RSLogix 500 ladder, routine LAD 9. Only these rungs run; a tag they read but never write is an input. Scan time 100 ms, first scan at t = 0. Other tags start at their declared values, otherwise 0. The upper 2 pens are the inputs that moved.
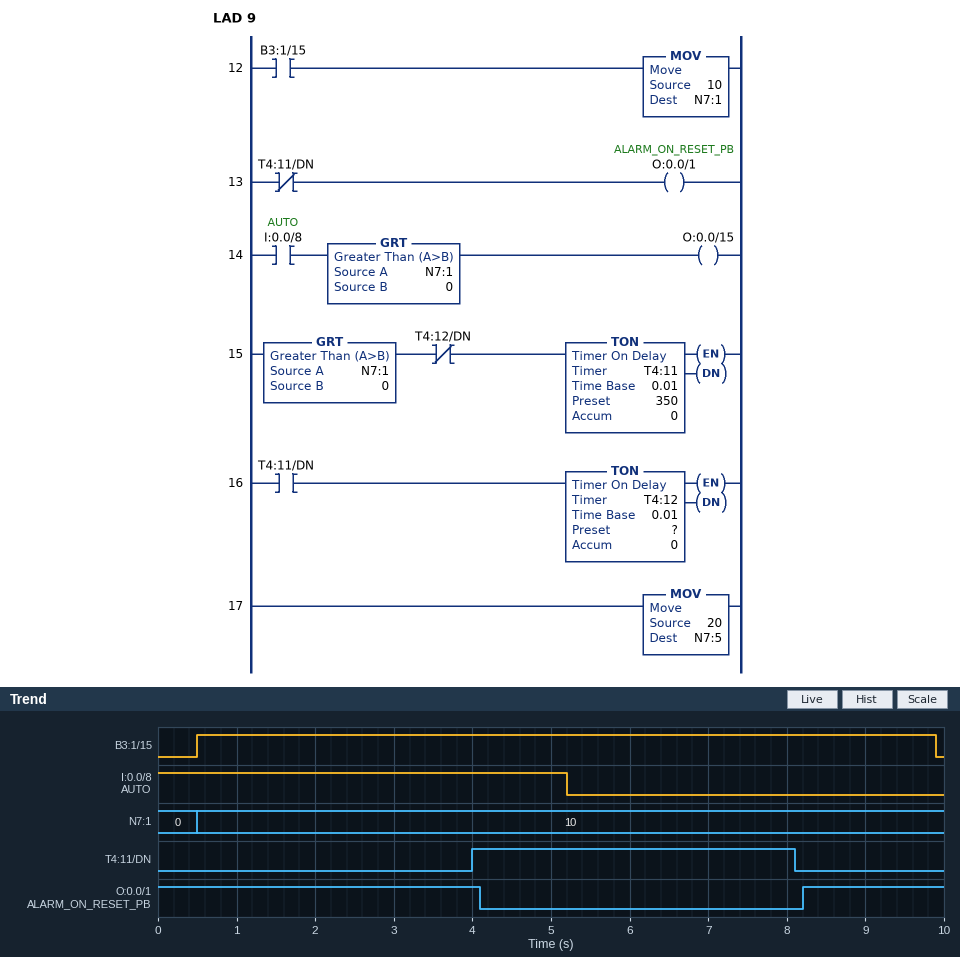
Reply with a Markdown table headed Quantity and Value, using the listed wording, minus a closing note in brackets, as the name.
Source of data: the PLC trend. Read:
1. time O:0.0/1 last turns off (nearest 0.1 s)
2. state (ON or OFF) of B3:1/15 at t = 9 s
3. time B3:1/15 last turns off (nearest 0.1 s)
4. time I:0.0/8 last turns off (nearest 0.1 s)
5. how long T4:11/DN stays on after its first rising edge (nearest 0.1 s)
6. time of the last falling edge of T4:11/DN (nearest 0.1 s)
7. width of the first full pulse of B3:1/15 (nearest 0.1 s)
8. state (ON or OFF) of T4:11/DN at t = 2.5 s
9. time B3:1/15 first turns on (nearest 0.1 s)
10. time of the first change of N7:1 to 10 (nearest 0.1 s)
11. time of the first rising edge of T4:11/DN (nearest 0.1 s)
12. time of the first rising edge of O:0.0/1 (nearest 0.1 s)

| Quantity | Value |
|---|---|
| time O:0.0/1 last turns off | 4.1 s |
| state (ON or OFF) of B3:1/15 at t = 9 s | ON |
| time B3:1/15 last turns off | 9.9 s |
| time I:0.0/8 last turns off | 5.2 s |
| how long T4:11/DN stays on after its first rising edge | 4.1 s |
| time of the last falling edge of T4:11/DN | 8.1 s |
| width of the first full pulse of B3:1/15 | 9.4 s |
| state (ON or OFF) of T4:11/DN at t = 2.5 s | OFF |
| time B3:1/15 first turns on | 0.5 s |
| time of the first change of N7:1 to 10 | 0.5 s |
| time of the first rising edge of T4:11/DN | 4.0 s |
| time of the first rising edge of O:0.0/1 | 8.2 s |
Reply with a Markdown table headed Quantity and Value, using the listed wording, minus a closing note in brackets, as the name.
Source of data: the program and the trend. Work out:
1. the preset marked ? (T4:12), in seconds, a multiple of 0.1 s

| Quantity | Value |
|---|---|
| the preset marked ? (T4:12), in seconds, a multiple of 0.1 s | 4.0 s |
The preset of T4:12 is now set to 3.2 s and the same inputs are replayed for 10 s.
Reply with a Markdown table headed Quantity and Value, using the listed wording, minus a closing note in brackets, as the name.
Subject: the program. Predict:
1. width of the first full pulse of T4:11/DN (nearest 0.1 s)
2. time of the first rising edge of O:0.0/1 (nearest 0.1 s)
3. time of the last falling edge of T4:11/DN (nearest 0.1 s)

| Quantity | Value |
|---|---|
| width of the first full pulse of T4:11/DN | 3.3 s |
| time of the first rising edge of O:0.0/1 | 7.4 s |
| time of the last falling edge of T4:11/DN | 7.3 s |
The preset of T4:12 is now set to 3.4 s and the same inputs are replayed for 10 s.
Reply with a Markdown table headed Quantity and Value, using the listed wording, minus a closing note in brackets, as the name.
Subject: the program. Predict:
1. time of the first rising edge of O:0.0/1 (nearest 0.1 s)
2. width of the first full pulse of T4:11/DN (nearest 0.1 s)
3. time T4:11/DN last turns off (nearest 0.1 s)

| Quantity | Value |
|---|---|
| time of the first rising edge of O:0.0/1 | 7.6 s |
| width of the first full pulse of T4:11/DN | 3.5 s |
| time T4:11/DN last turns off | 7.5 s |
